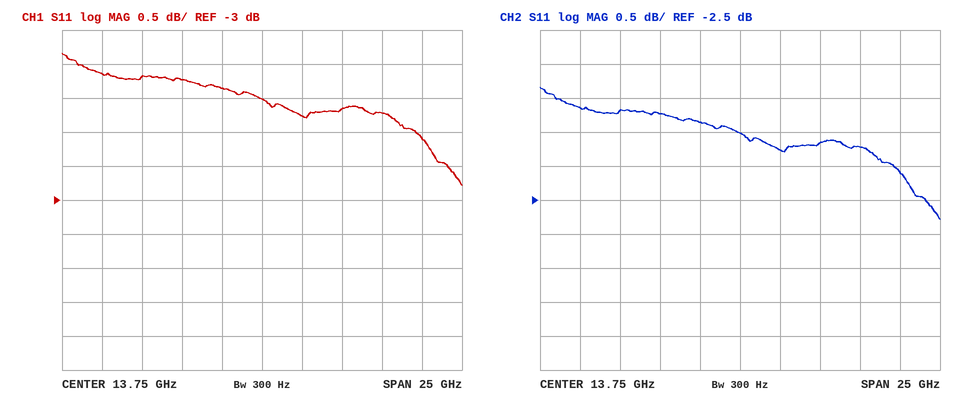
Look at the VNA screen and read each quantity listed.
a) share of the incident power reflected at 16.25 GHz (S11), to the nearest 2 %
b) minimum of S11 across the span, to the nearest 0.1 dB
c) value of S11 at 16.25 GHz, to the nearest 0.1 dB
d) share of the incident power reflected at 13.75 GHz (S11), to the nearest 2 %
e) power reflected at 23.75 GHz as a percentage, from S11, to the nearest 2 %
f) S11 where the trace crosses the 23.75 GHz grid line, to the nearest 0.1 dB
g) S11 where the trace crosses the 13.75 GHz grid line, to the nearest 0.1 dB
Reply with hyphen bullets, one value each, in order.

- 66 %
- -2.8 dB
- -1.8 dB
- 70 %
- 62 %
- -2.1 dB
- -1.5 dB
